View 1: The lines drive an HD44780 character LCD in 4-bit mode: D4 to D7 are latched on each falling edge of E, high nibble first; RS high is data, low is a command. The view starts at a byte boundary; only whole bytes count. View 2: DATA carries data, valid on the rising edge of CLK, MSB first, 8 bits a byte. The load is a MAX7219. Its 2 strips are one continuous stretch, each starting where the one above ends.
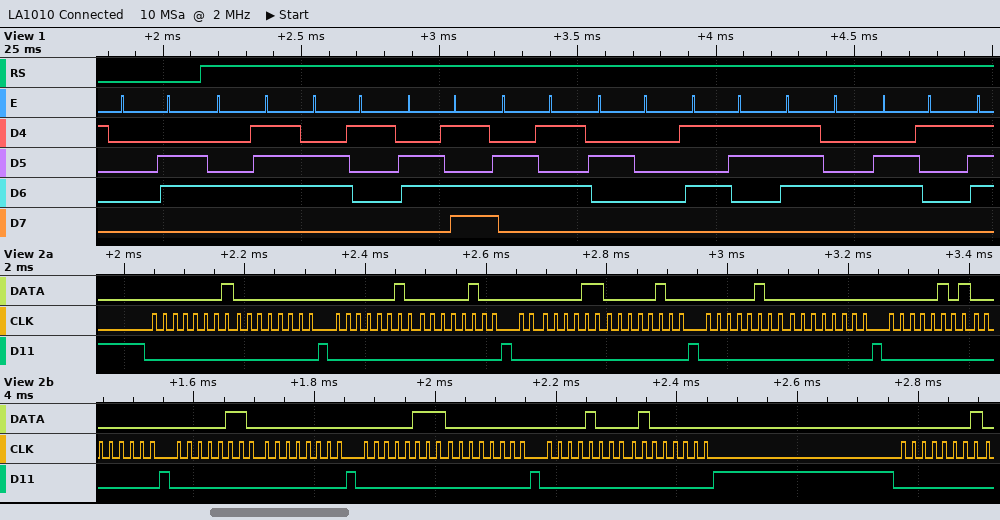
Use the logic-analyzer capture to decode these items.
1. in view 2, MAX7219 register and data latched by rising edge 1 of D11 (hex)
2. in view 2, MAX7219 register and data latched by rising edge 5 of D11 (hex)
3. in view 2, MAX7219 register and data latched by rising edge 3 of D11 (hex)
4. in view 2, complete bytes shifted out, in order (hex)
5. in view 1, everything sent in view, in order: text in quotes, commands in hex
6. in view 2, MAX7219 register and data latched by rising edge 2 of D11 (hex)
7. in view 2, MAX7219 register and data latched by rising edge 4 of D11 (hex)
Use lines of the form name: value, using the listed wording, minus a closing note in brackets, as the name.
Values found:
in view 2, MAX7219 register and data latched by rising edge 1 of D11: register 0x1, data 0x00
in view 2, MAX7219 register and data latched by rising edge 5 of D11: register 0x5, data 0x00
in view 2, MAX7219 register and data latched by rising edge 3 of D11: register 0x3, data 0x04
in view 2, complete bytes shifted out, in order: 01 00 02 04 03 04 04 00 05 00 06 00 07 00 08 40 01
in view 1, everything sent in view, in order: text in quotes, commands in hex: 0x06 "Game Sta"
in view 2, MAX7219 register and data latched by rising edge 2 of D11: register 0x2, data 0x04
in view 2, MAX7219 register and data latched by rising edge 4 of D11: register 0x4, data 0x00
